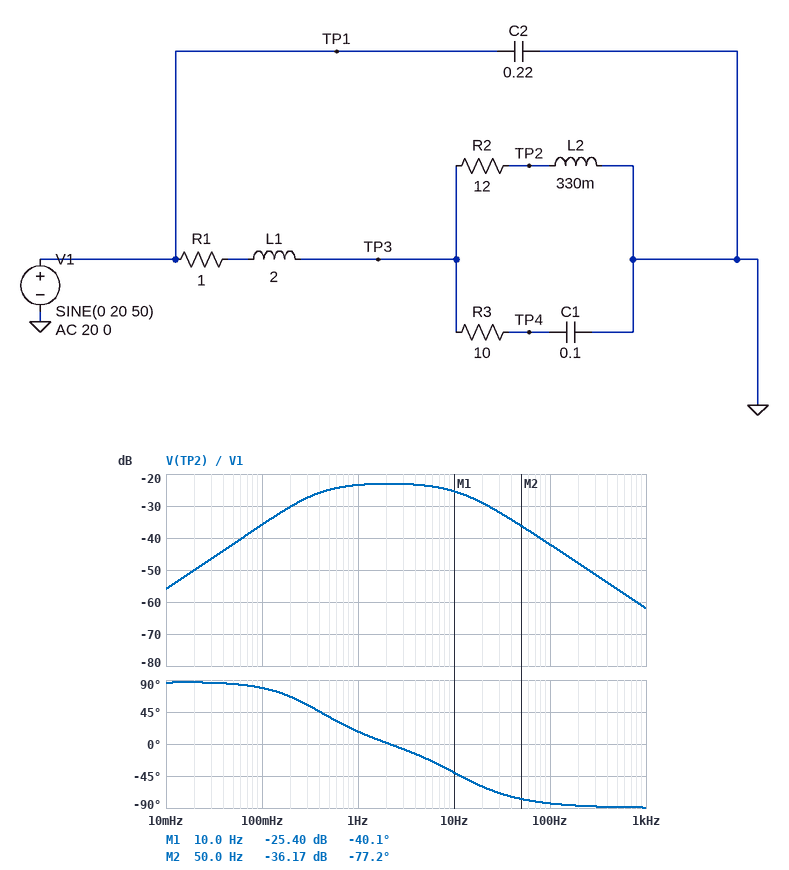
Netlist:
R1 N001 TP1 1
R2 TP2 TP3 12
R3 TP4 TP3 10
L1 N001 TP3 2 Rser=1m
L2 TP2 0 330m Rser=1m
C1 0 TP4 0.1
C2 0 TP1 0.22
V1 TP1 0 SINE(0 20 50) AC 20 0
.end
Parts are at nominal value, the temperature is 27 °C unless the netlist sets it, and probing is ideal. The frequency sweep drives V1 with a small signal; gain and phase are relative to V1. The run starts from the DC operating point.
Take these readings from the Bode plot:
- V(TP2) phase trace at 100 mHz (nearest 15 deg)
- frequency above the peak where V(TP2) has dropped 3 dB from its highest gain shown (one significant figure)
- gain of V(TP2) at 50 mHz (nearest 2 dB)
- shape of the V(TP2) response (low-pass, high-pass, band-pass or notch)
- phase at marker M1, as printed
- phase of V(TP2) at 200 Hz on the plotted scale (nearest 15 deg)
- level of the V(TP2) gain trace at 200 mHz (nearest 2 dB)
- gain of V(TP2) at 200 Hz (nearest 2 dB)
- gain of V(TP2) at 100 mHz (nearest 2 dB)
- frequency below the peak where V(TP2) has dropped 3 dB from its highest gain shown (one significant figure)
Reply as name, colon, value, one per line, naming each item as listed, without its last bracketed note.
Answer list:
V(TP2) phase trace at 100 mHz: 75 deg
frequency above the peak where V(TP2) has dropped 3 dB from its highest gain shown: 10 Hz
gain of V(TP2) at 50 mHz: -42 dB
shape of the V(TP2) response: band-pass
phase at marker M1, as printed: -40.1 deg
phase of V(TP2) at 200 Hz on the plotted scale: -90 deg
level of the V(TP2) gain trace at 200 mHz: -30 dB
gain of V(TP2) at 200 Hz: -48 dB
gain of V(TP2) at 100 mHz: -36 dB
frequency below the peak where V(TP2) has dropped 3 dB from its highest gain shown: 400 mHz
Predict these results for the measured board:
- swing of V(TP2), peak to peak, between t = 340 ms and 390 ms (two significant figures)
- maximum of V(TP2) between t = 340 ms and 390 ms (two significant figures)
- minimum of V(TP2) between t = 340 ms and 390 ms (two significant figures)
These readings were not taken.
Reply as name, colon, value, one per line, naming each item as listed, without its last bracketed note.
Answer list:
swing of V(TP2), peak to peak, between t = 340 ms and 390 ms: 620 mV
maximum of V(TP2) between t = 340 ms and 390 ms: 310 mV
minimum of V(TP2) between t = 340 ms and 390 ms: -320 mV
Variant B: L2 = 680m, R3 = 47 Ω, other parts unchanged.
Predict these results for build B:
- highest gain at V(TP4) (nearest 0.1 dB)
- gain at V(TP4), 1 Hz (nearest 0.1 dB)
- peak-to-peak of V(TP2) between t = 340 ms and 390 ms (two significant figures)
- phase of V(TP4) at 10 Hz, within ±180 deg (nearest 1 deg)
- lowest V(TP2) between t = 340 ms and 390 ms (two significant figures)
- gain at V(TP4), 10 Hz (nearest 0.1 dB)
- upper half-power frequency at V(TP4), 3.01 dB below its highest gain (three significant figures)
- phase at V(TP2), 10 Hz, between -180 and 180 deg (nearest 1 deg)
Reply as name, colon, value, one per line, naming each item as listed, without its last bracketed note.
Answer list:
highest gain at V(TP4): -0.7 dB
gain at V(TP4), 1 Hz: -34.7 dB
peak-to-peak of V(TP2) between t = 340 ms and 390 ms: 2.8 V
phase of V(TP4) at 10 Hz, within ±180 deg: -132 deg
lowest V(TP2) between t = 340 ms and 390 ms: -1.4 V
gain at V(TP4), 10 Hz: -63.5 dB
upper half-power frequency at V(TP4), 3.01 dB below its highest gain: 33.4 mHz
phase at V(TP2), 10 Hz, between -180 and 180 deg: -27 deg
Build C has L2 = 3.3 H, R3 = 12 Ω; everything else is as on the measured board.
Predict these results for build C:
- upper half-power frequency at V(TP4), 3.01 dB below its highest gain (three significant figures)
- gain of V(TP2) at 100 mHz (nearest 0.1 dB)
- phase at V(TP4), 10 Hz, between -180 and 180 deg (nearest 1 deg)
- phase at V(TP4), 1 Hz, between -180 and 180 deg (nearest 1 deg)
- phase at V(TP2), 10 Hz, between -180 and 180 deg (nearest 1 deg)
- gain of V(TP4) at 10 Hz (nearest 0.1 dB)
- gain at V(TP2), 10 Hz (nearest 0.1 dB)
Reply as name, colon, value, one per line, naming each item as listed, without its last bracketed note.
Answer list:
upper half-power frequency at V(TP4), 3.01 dB below its highest gain: 128 mHz
gain of V(TP2) at 100 mHz: -16.1 dB
phase at V(TP4), 10 Hz, between -180 and 180 deg: -171 deg
phase at V(TP4), 1 Hz, between -180 and 180 deg: -124 deg
phase at V(TP2), 10 Hz, between -180 and 180 deg: -78 deg
gain of V(TP4) at 10 Hz: -58.1 dB
gain at V(TP2), 10 Hz: -20.5 dB
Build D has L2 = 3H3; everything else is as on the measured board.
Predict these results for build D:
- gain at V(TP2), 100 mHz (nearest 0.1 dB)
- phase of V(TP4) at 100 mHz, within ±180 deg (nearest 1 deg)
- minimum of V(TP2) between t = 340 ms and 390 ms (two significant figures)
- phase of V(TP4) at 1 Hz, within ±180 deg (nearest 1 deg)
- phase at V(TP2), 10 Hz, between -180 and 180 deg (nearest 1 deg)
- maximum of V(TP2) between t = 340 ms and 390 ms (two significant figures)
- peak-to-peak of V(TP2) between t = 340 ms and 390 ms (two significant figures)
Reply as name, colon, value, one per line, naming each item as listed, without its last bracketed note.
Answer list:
gain at V(TP2), 100 mHz: -16.1 dB
phase of V(TP4) at 100 mHz, within ±180 deg: -41 deg
minimum of V(TP2) between t = 340 ms and 390 ms: -350 mV
phase of V(TP4) at 1 Hz, within ±180 deg: -128 deg
phase at V(TP2), 10 Hz, between -180 and 180 deg: -80 deg
maximum of V(TP2) between t = 340 ms and 390 ms: 290 mV
peak-to-peak of V(TP2) between t = 340 ms and 390 ms: 640 mV
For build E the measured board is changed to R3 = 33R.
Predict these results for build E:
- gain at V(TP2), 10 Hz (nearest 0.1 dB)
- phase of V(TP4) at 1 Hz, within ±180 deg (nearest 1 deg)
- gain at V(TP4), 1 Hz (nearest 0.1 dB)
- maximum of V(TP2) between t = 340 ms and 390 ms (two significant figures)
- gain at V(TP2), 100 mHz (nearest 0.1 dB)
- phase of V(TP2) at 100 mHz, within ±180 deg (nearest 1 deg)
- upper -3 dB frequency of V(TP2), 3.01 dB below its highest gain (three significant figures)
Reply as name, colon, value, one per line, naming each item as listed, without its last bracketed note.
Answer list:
gain at V(TP2), 10 Hz: -19.8 dB
phase of V(TP4) at 1 Hz, within ±180 deg: -135 deg
gain at V(TP4), 1 Hz: -31.8 dB
maximum of V(TP2) between t = 340 ms and 390 ms: 940 mV
gain at V(TP2), 100 mHz: -36.1 dB
phase of V(TP2) at 100 mHz, within ±180 deg: 81 deg
upper -3 dB frequency of V(TP2), 3.01 dB below its highest gain: 25.0 Hz
